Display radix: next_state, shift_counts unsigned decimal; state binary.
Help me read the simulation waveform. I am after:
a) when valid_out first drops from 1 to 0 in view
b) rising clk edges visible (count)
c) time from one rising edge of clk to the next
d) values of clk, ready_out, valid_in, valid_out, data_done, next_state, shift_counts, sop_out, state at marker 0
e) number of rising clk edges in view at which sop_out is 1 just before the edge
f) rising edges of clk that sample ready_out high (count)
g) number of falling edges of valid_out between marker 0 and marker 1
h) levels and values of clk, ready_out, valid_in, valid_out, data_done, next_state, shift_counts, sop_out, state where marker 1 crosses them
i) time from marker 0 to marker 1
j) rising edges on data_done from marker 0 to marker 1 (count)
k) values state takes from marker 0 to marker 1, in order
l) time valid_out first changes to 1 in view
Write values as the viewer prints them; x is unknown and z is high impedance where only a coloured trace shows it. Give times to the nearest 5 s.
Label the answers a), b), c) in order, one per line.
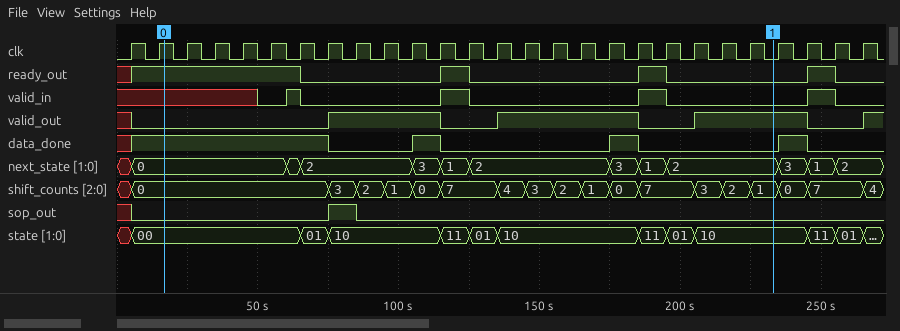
a) 115 s
b) 27
c) 10 s
d) clk=1, ready_out=1, valid_in=x, valid_out=0, data_done=1, next_state=0, shift_counts=0, sop_out=0, state=00
e) 1
f) 9
g) 2
h) clk=0, ready_out=0, valid_in=0, valid_out=1, data_done=0, next_state=2, shift_counts=1, sop_out=0, state=10
i) 215 s
j) 2
k) 00, 01, 10, 11, 01, 10, 11, 01, 10
l) 75 s
